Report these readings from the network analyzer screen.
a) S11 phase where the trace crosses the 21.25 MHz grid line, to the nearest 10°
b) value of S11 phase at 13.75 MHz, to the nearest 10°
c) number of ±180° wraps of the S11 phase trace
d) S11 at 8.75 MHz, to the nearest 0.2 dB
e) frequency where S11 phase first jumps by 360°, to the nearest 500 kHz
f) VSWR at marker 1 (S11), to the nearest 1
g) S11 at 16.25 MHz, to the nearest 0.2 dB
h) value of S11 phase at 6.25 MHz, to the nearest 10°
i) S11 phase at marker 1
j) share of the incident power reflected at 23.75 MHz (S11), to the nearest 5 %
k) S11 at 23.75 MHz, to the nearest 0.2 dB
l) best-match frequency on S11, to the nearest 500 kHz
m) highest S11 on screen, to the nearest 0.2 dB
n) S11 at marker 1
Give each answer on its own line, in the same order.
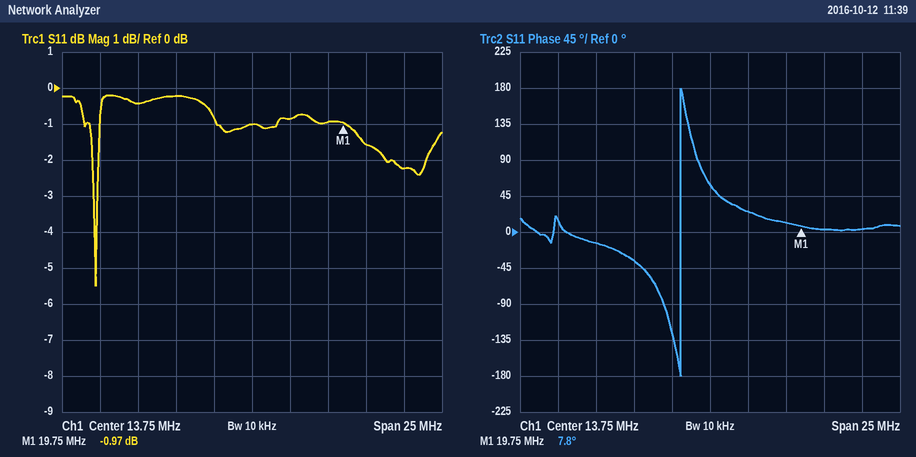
0°
60°
1
-0.2 dB
12.0 MHz
18
-0.8 dB
-10°
7.8°
60 %
-2.2 dB
3.5 MHz
-0.2 dB
-0.97 dB
